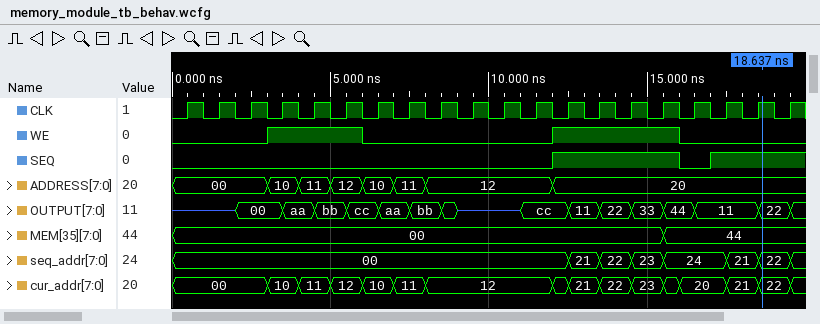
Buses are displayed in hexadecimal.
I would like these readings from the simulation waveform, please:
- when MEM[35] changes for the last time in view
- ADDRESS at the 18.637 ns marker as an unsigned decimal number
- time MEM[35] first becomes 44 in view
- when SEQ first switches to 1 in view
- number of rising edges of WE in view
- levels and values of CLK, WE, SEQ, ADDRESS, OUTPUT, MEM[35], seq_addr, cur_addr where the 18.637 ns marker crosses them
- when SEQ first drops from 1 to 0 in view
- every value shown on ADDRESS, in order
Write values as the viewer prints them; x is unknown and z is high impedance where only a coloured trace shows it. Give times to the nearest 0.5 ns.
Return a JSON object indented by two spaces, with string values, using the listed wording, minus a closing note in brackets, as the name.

{
  "when MEM[35] changes for the last time in view": "15.5 ns",
  "ADDRESS at the 18.637 ns marker as an unsigned decimal number": "32",
  "time MEM[35] first becomes 44 in view": "15.5 ns",
  "when SEQ first switches to 1 in view": "12 ns",
  "number of rising edges of WE in view": "2",
  "levels and values of CLK, WE, SEQ, ADDRESS, OUTPUT, MEM[35], seq_addr, cur_addr where the 18.637 ns marker crosses them": "CLK=1, WE=0, SEQ=1, ADDRESS=20, OUTPUT=22, MEM[35]=44, seq_addr=22, cur_addr=22",
  "when SEQ first drops from 1 to 0 in view": "16 ns",
  "every value shown on ADDRESS, in order": "00, 10, 11, 12, 10, 11, 12, 20"
}
